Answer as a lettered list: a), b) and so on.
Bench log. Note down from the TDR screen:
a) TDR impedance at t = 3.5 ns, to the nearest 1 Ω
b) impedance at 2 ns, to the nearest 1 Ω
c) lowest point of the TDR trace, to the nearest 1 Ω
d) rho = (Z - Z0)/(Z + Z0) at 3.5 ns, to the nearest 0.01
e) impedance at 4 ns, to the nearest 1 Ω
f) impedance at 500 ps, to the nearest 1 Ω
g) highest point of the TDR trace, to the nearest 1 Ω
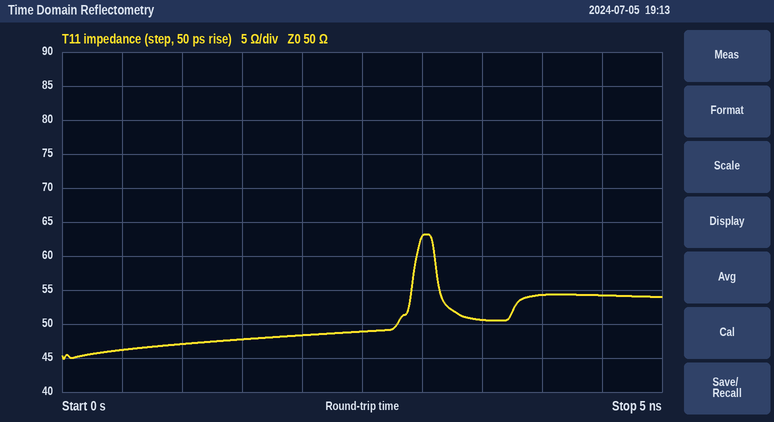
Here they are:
a) 51 Ω
b) 48 Ω
c) 45 Ω
d) +0.01
e) 54 Ω
f) 46 Ω
g) 63 Ω
